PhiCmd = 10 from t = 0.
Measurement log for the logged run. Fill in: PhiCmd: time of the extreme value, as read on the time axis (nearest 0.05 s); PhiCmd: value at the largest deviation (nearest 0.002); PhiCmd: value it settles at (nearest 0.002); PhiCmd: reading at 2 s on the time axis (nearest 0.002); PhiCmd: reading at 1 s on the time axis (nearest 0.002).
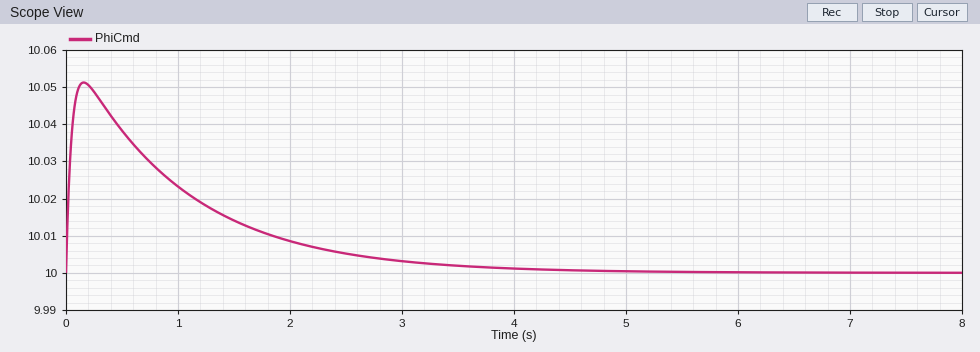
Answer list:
0.15 s
10.052
10.000
10.008
10.024
